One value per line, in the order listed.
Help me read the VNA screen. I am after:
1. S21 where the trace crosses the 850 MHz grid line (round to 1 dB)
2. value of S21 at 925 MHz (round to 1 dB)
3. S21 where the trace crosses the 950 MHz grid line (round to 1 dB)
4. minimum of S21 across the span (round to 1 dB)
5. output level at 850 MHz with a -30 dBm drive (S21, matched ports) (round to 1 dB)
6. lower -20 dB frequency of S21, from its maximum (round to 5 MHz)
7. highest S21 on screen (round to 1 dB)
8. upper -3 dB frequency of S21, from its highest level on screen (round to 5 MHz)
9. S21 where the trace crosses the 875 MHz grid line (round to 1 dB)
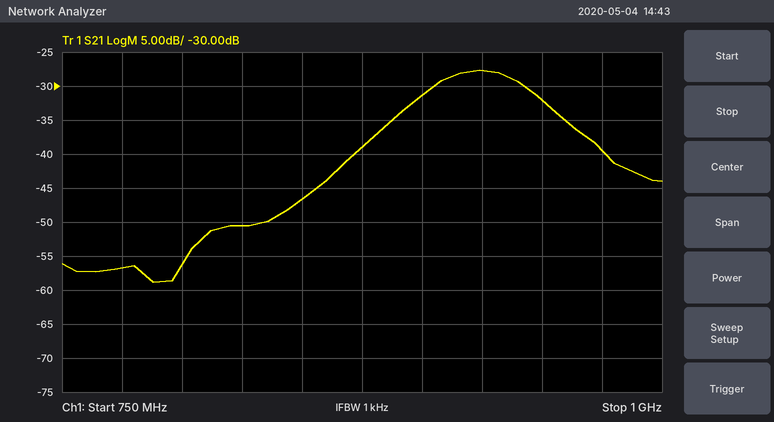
-47 dB
-28 dB
-32 dB
-59 dB
-77 dBm
845 MHz
-28 dB
945 MHz
-39 dB
